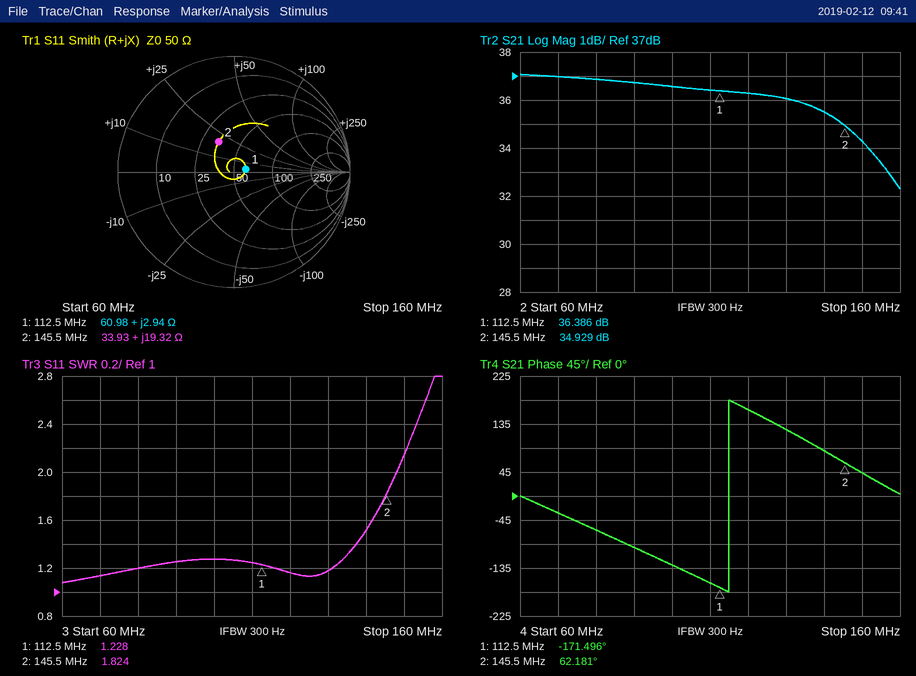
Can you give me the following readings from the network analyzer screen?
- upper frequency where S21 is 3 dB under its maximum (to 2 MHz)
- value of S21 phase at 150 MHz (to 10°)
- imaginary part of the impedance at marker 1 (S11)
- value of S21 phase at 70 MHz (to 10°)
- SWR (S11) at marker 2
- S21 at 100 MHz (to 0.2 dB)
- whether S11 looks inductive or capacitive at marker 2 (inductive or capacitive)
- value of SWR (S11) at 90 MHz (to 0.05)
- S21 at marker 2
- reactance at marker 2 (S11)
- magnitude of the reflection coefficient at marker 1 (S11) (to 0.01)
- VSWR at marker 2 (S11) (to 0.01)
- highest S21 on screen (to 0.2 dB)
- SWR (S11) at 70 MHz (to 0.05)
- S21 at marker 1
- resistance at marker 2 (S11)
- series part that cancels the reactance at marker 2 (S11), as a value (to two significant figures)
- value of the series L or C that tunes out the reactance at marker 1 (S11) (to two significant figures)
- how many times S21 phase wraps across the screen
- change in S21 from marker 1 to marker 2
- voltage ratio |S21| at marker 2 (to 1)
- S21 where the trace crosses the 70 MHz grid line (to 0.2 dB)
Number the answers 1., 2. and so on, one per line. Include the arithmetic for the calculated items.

1. 152 MHz
2. 40°
3. +2.94 Ω
4. -30°
5. 1.824
6. 36.6 dB
7. inductive
8. 1.25
9. 34.929 dB
10. +19.32 Ω
11. 0.10
12. 1.82
13. 37.0 dB
14. 1.15
15. 36.386 dB
16. 33.93 Ω
17. C = 1/(2π × 145.5 MHz × 19.32 Ω) ≈ 57 pF
18. C = 1/(2π × 112.5 MHz × 2.94 Ω) ≈ 481 pF, so 480 pF to two significant figures
19. 1
20. 34.929 − (36.386) = -1.457 dB
21. 10^(34.929/20) ≈ 56
22. 37.0 dB
